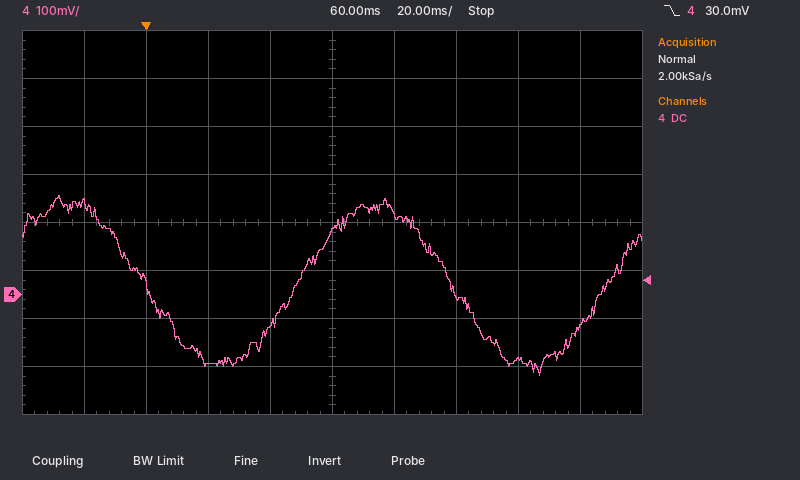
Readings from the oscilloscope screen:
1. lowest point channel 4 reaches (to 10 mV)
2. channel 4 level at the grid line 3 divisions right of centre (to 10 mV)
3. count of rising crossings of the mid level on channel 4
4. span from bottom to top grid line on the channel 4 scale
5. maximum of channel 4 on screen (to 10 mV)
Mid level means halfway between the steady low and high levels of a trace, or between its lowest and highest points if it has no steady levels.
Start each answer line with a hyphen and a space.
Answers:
- -170 mV
- -130 mV
- 2
- 800 mV
- 210 mV
